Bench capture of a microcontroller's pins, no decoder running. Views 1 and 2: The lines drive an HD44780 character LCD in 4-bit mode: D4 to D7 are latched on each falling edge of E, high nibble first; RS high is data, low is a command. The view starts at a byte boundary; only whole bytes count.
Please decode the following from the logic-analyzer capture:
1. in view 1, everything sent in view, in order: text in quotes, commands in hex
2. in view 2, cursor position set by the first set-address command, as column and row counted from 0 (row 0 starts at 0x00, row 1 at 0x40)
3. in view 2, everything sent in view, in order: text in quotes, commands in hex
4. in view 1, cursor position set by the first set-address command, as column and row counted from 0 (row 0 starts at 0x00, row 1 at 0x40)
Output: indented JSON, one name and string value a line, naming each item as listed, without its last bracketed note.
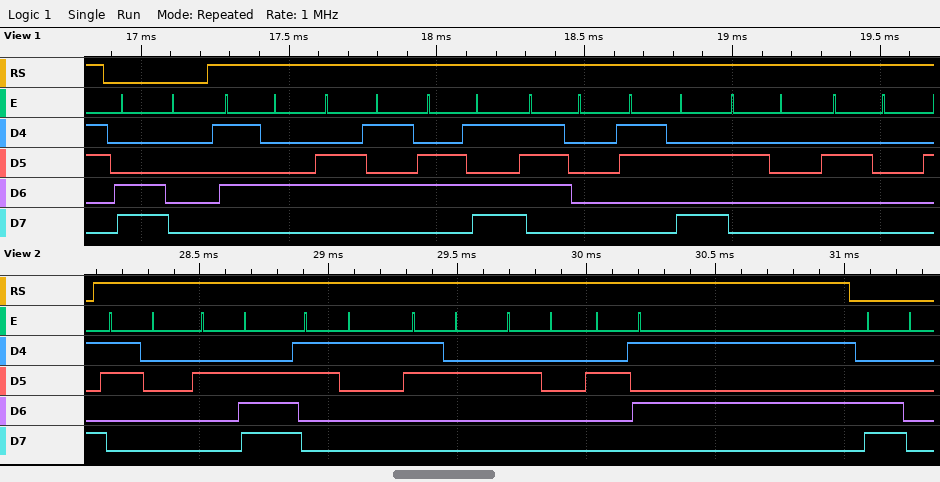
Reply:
{
  "in view 1, everything sent in view, in order: text in quotes, commands in hex": "0xC0 \"Temp:  \"",
  "in view 2, cursor position set by the first set-address command, as column and row counted from 0": "column 0, row 1",
  "in view 2, everything sent in view, in order: text in quotes, commands in hex": "\"0.12 %\" 0xC0",
  "in view 1, cursor position set by the first set-address command, as column and row counted from 0": "column 0, row 1"
}
